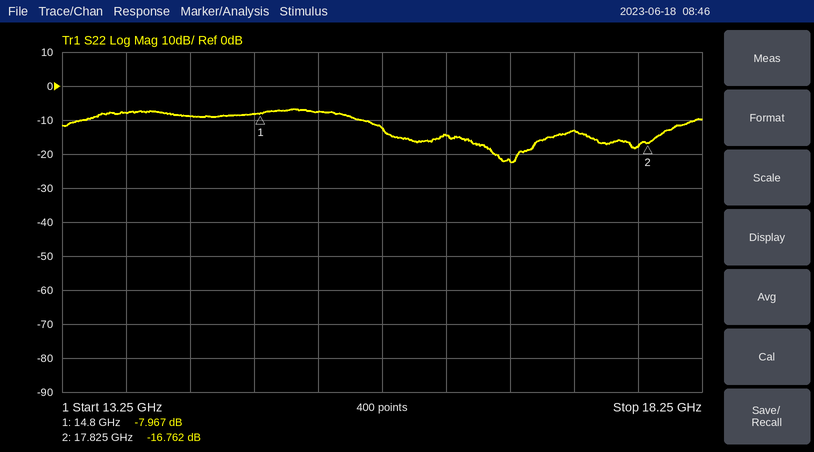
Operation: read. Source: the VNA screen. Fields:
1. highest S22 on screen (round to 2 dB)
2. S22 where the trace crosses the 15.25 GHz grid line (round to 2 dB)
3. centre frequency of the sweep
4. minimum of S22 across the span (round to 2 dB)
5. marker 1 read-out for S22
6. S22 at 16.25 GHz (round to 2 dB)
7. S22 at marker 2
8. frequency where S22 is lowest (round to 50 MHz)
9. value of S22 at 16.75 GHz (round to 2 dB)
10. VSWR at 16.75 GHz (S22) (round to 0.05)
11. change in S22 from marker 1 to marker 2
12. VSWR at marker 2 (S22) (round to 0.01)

-6 dB
-8 dB
15.75 GHz
-22 dB
-7.967 dB
-14 dB
-16.762 dB
16.75 GHz
-22 dB
1.15
-8.795 dB
1.34
